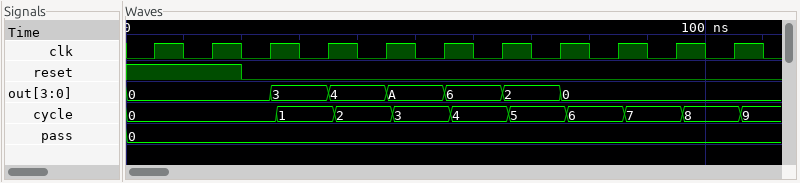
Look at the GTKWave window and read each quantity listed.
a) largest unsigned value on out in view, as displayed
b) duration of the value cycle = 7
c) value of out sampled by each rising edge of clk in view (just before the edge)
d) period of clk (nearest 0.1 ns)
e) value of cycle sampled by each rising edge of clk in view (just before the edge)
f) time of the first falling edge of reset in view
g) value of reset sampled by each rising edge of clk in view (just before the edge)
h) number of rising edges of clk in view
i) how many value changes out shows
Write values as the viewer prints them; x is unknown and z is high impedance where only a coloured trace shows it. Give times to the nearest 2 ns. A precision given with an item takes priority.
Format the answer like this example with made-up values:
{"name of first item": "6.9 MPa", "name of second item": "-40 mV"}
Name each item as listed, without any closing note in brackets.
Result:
{"largest unsigned value on out in view, as displayed": "A", "duration of the value cycle = 7": "10 ns", "value of out sampled by each rising edge of clk in view": "0, 0, 0, 3, 4, A, 6, 2, 0, 0, 0", "period of clk": "10 ns", "value of cycle sampled by each rising edge of clk in view": "0, 0, 0, 1, 2, 3, 4, 5, 6, 7, 8", "time of the first falling edge of reset in view": "20 ns", "value of reset sampled by each rising edge of clk in view": "1 1 0 0 0 0 0 0 0 0 0", "number of rising edges of clk in view": "11", "how many value changes out shows": "6"}
